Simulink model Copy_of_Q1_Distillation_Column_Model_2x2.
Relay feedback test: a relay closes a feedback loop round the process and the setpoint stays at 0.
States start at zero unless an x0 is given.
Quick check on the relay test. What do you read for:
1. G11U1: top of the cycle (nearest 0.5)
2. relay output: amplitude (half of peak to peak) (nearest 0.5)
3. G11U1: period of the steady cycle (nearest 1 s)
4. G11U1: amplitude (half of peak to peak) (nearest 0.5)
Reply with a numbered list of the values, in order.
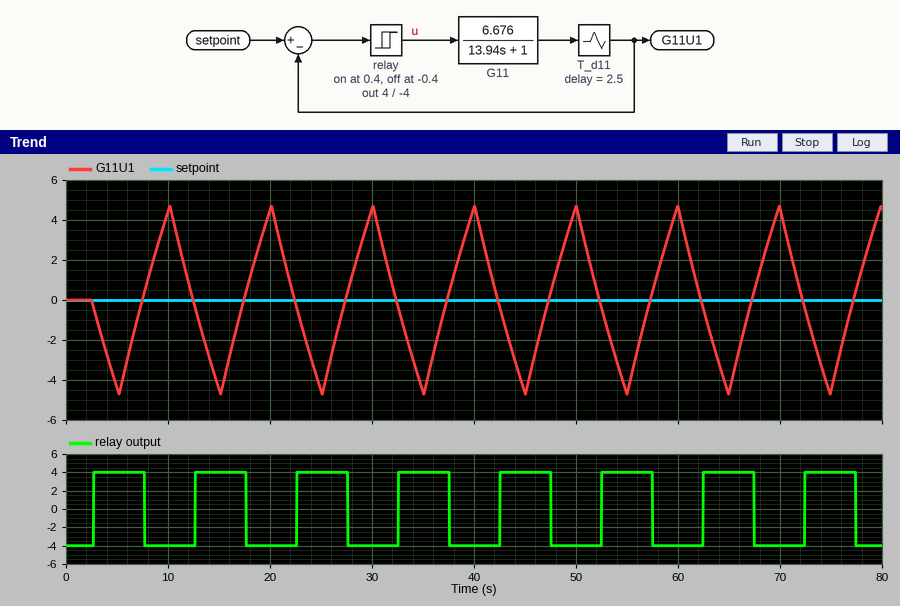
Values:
1. 4.5
2. 4.0
3. 10 s
4. 4.5
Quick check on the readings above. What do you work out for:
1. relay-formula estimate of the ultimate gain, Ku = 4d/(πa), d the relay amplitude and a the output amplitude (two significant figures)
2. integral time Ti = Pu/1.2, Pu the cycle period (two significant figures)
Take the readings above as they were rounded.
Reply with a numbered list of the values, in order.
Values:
1. 1.1
2. 8.3 s
